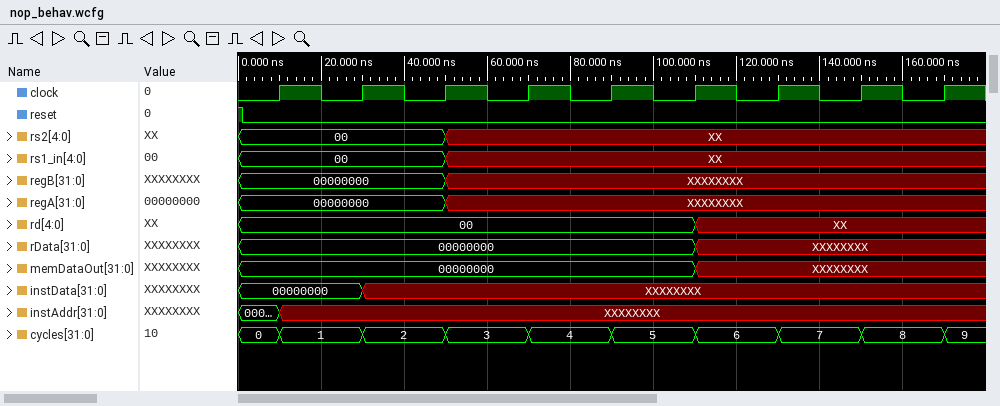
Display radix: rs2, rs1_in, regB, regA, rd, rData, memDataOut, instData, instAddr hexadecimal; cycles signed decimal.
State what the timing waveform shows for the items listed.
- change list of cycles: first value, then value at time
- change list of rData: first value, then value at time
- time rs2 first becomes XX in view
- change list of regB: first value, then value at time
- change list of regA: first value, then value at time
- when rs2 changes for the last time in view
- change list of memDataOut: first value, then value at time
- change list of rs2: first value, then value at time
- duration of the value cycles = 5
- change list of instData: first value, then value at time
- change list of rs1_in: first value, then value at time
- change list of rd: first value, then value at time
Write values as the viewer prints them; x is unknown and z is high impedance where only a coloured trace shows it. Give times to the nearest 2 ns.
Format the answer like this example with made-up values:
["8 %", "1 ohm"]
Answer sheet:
["0, 1 at 10 ns, 2 at 30 ns, 3 at 50 ns, 4 at 70 ns, 5 at 90 ns, 6 at 110 ns, 7 at 130 ns, 8 at 150 ns, 9 at 170 ns", "00000000, XXXXXXXX at 110 ns", "50 ns", "00000000, XXXXXXXX at 50 ns", "00000000, XXXXXXXX at 50 ns", "50 ns", "00000000, XXXXXXXX at 110 ns", "00, XX at 50 ns", "20 ns", "00000000, XXXXXXXX at 30 ns", "00, XX at 50 ns", "00, XX at 110 ns"]
